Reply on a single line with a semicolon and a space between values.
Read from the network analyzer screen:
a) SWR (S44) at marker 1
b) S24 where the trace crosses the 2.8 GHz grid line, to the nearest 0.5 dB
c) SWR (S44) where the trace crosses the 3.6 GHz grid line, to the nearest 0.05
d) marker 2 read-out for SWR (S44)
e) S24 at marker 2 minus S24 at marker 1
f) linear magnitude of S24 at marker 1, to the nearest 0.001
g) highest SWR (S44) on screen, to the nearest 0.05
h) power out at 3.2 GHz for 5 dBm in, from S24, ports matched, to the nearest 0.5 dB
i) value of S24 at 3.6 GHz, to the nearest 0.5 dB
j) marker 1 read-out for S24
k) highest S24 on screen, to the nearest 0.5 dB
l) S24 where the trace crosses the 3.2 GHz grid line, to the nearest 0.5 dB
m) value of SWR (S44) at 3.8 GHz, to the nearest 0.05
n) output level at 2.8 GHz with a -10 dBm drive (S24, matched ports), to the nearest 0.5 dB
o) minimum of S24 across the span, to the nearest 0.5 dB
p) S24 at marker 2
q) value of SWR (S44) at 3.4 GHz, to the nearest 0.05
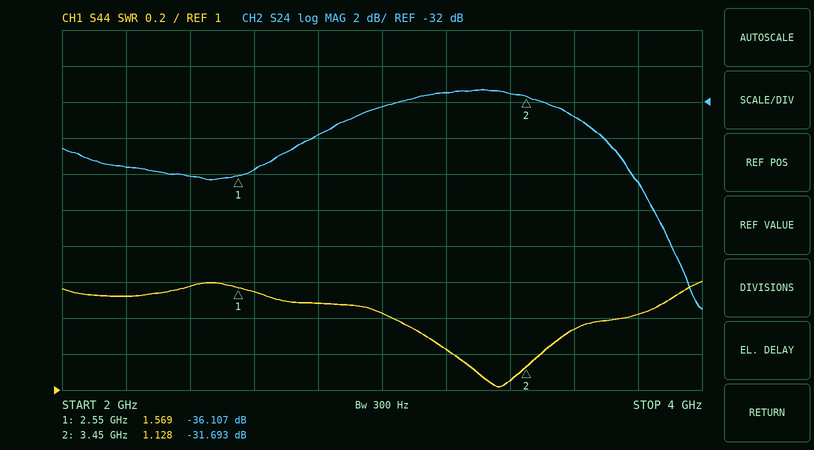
1.569; -34.0 dB; 1.35; 1.128; 4.414 dB; 0.016; 1.60; -26.5 dBm; -33.0 dB; -36.107 dB; -31.5 dB; -31.5 dB; 1.40; -44.0 dBm; -43.5 dB; -31.693 dB; 1.05
